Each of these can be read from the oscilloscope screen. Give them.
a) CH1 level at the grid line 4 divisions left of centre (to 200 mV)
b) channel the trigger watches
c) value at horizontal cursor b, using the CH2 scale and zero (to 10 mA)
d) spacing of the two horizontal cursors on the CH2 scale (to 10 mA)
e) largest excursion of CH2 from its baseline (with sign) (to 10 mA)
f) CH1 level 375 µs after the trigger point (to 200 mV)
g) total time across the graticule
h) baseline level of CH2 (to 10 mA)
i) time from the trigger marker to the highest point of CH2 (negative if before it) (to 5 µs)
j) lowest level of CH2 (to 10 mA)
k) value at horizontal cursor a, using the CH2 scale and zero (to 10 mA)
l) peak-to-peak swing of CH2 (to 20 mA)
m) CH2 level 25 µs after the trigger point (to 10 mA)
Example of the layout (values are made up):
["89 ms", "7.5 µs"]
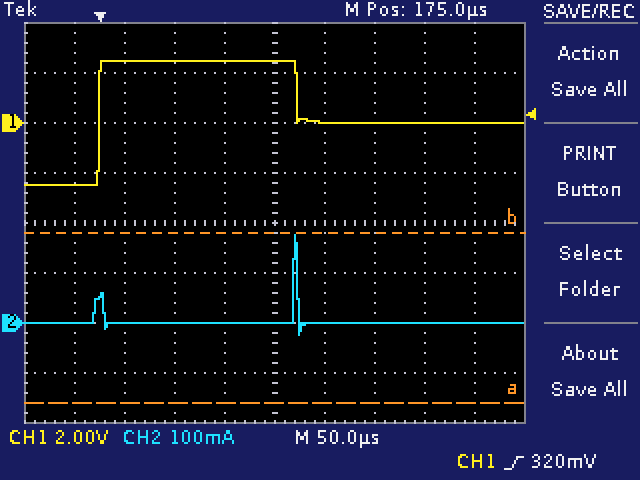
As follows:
["-2.4 V", "CH1", "180 mA", "340 mA", "+180 mA", "0.0 V", "500 µs", "0 mA", "+195 µs", "-20 mA", "-160 mA", "200 mA", "0 mA"]
